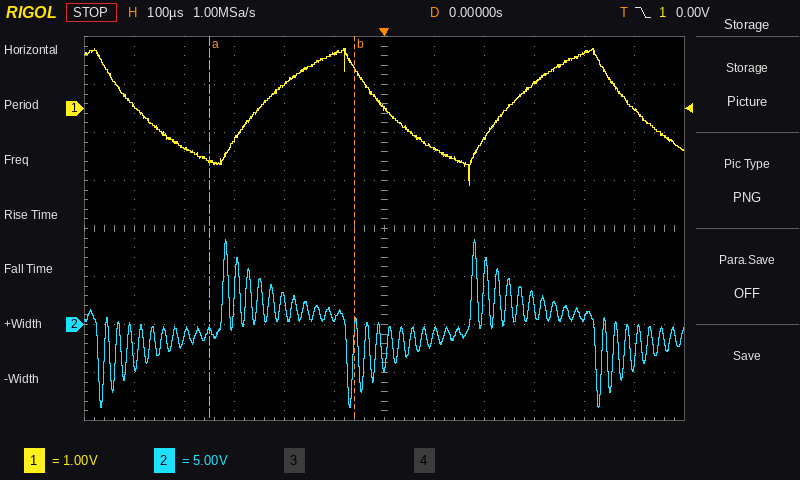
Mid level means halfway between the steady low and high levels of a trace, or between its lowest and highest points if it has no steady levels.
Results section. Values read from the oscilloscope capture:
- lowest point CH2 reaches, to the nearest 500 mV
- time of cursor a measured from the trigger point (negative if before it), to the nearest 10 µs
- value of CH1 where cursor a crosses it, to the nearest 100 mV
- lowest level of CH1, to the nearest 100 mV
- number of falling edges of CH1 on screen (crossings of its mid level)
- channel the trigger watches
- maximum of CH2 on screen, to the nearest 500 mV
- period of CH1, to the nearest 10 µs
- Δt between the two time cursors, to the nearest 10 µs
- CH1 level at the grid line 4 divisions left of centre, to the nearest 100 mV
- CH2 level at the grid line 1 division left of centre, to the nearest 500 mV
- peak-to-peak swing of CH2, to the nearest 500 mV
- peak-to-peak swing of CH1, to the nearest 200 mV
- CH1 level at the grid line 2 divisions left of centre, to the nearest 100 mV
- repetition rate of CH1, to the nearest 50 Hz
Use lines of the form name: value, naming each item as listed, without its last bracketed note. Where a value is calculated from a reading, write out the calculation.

lowest point CH2 reaches, to the nearest 500 mV: -8.5 V
time of cursor a measured from the trigger point (negative if before it), to the nearest 10 µs: -350 µs
value of CH1 where cursor a crosses it, to the nearest 100 mV: -1.1 V
lowest level of CH1, to the nearest 100 mV: -1.6 V
number of falling edges of CH1 on screen: 3
channel the trigger watches: CH1
maximum of CH2 on screen, to the nearest 500 mV: 9.0 V
period of CH1, to the nearest 10 µs: 500 µs
Δt between the two time cursors, to the nearest 10 µs: 290 µs
CH1 level at the grid line 4 divisions left of centre, to the nearest 100 mV: -800 mV
CH2 level at the grid line 1 division left of centre, to the nearest 500 mV: 500 mV
peak-to-peak swing of CH2, to the nearest 500 mV: 9.0 V − (-8.5 V) = 17.5 V
peak-to-peak swing of CH1, to the nearest 200 mV: 2.8 V
CH1 level at the grid line 2 divisions left of centre, to the nearest 100 mV: 500 mV
repetition rate of CH1, to the nearest 50 Hz: 1 / 500 µs ≈ 2.00 kHz
